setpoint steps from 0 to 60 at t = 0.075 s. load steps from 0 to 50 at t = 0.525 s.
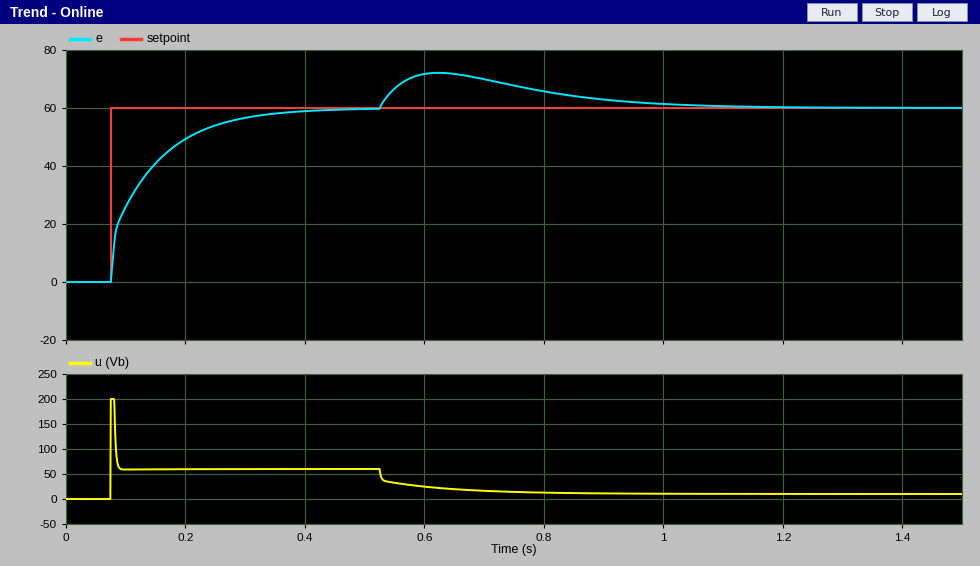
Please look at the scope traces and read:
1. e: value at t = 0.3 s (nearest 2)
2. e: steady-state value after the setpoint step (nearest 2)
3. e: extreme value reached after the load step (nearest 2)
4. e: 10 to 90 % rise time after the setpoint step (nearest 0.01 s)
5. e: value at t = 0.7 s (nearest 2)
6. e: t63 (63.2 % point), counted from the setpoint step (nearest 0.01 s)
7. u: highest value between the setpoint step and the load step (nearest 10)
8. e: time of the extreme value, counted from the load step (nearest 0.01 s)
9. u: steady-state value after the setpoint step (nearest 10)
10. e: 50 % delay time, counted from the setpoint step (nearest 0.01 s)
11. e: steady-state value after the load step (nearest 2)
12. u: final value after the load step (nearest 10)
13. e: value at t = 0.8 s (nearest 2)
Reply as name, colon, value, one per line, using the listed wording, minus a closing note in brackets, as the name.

e: value at t = 0.3 s: 56
e: steady-state value after the setpoint step: 60
e: extreme value reached after the load step: 72
e: 10 to 90 % rise time after the setpoint step: 0.17 s
e: value at t = 0.7 s: 70
e: t63 (63.2 % point), counted from the setpoint step: 0.06 s
u: highest value between the setpoint step and the load step: 200
e: time of the extreme value, counted from the load step: 0.10 s
u: steady-state value after the setpoint step: 60
e: 50 % delay time, counted from the setpoint step: 0.04 s
e: steady-state value after the load step: 60
u: final value after the load step: 10
e: value at t = 0.8 s: 66
